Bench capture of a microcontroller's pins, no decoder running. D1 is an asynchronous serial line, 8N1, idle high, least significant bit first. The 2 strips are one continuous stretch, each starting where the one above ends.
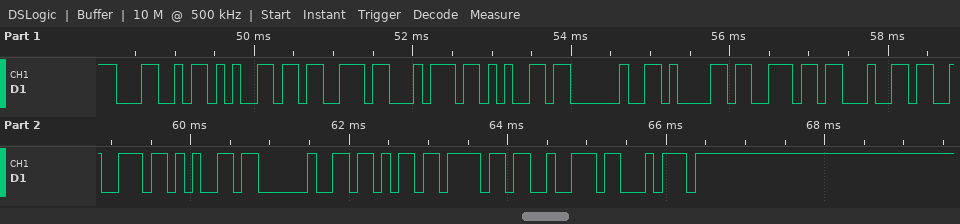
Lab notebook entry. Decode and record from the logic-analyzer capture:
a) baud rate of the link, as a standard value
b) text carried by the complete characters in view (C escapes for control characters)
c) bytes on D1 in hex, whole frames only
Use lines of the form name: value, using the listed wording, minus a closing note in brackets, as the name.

baud rate of the link, as a standard value: 9600 baud
text carried by the complete characters in view: "Leste andre kort"
bytes on D1 in hex, whole frames only: 4C 65 73 74 65 20 61 6E 64 72 65 20 6B 6F 72 74
